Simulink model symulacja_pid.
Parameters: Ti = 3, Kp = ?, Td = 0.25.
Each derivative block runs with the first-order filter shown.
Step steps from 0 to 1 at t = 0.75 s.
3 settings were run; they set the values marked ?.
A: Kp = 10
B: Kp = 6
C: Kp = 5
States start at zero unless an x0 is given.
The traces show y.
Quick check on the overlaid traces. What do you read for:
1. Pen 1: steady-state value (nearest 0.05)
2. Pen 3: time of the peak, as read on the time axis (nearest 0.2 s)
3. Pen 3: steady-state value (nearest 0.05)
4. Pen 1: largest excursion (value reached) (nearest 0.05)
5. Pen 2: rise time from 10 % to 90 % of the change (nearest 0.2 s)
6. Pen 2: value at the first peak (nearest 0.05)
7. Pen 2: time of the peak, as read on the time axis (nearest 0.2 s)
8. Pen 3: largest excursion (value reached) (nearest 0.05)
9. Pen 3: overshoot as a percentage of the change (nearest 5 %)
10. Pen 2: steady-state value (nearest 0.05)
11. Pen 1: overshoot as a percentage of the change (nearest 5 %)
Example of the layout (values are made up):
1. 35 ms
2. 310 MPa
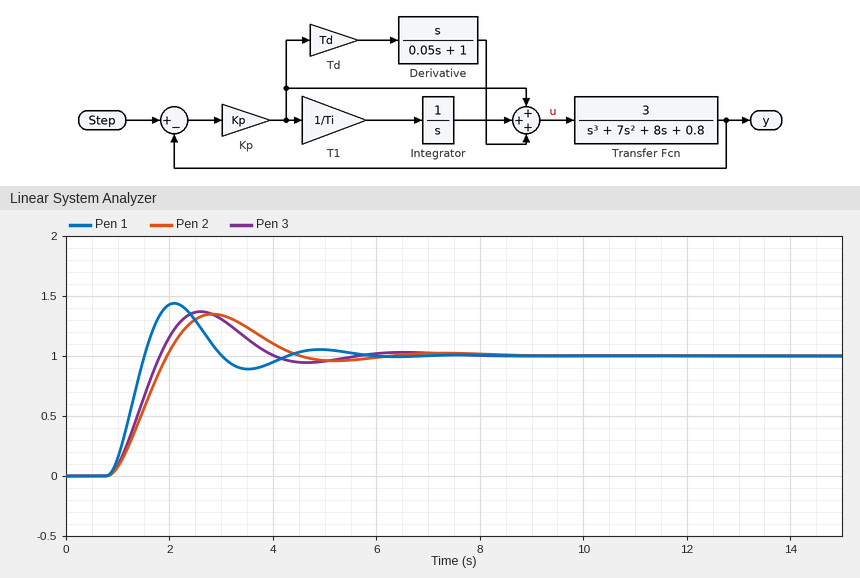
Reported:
1. 1.00
2. 2.6 s
3. 1.00
4. 1.45
5. 0.8 s
6. 1.35
7. 2.8 s
8. 1.35
9. 35 %
10. 1.00
11. 45 %
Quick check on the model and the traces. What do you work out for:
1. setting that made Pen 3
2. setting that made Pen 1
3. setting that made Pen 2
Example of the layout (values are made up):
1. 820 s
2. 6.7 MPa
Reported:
1. B
2. A
3. C
